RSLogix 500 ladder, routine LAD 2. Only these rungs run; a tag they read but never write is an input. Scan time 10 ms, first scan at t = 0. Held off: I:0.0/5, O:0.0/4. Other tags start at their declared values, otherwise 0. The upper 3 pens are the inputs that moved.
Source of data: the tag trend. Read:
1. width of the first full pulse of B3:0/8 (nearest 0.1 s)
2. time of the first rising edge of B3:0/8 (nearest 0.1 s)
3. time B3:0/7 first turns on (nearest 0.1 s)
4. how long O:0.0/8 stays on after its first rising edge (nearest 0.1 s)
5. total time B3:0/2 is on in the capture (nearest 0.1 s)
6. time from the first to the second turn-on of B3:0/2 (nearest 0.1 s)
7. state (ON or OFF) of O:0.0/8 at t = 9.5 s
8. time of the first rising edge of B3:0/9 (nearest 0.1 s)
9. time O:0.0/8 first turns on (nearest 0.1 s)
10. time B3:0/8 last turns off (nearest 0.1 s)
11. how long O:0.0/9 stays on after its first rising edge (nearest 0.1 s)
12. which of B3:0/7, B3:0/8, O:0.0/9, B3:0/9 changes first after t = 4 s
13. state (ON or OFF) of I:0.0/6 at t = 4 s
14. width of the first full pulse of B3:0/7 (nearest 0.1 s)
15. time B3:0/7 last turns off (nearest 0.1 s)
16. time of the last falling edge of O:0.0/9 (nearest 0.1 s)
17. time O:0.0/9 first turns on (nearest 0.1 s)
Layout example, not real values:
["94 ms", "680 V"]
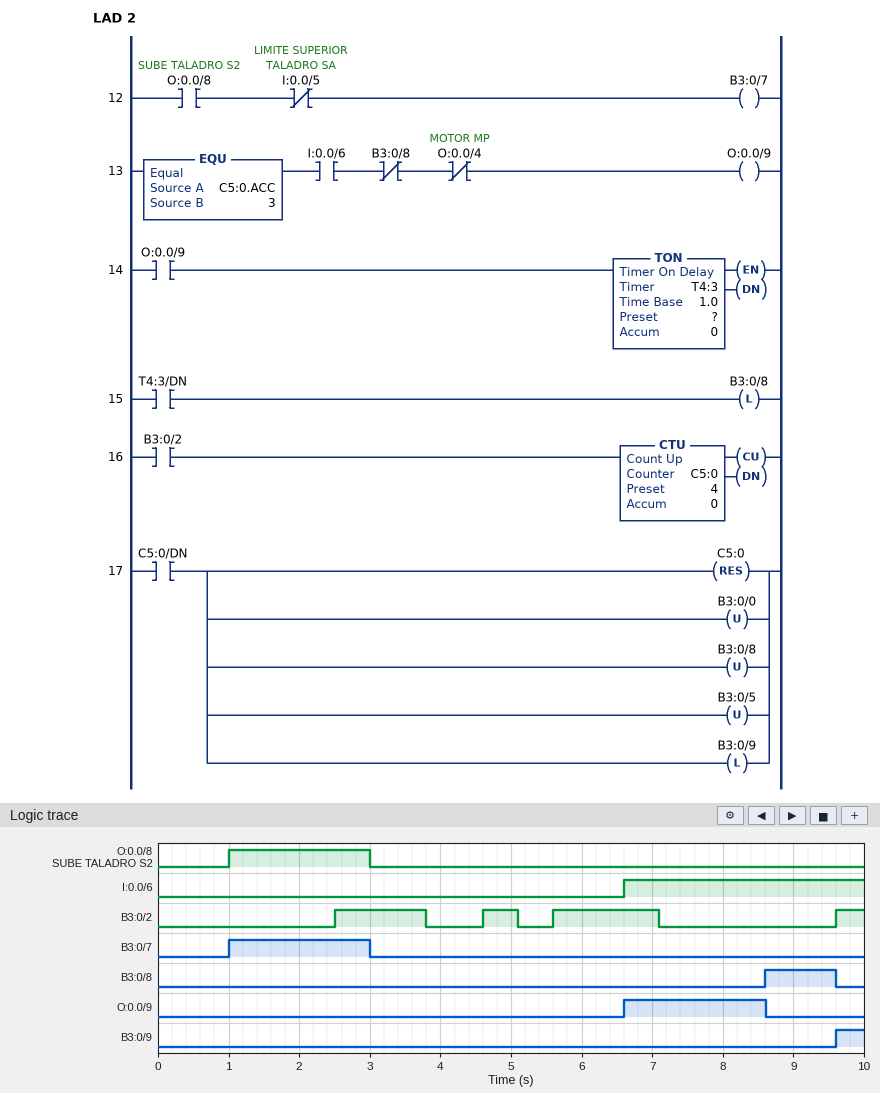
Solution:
["1.0 s", "8.6 s", "1.0 s", "2.0 s", "3.7 s", "2.1 s", "OFF", "9.6 s", "1.0 s", "9.6 s", "2.0 s", "O:0.0/9", "OFF", "2.0 s", "3.0 s", "8.6 s", "6.6 s"]
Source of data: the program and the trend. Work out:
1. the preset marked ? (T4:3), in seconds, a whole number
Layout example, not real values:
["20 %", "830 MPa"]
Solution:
["2 s"]
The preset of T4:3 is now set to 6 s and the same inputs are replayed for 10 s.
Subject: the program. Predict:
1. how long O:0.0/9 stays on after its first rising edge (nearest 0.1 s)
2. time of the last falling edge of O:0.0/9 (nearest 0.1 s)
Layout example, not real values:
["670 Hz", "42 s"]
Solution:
["3.0 s", "9.6 s"]
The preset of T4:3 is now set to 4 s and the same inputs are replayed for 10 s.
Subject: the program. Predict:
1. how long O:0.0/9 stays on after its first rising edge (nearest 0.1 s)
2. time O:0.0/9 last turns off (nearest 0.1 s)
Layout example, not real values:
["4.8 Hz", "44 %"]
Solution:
["3.0 s", "9.6 s"]
